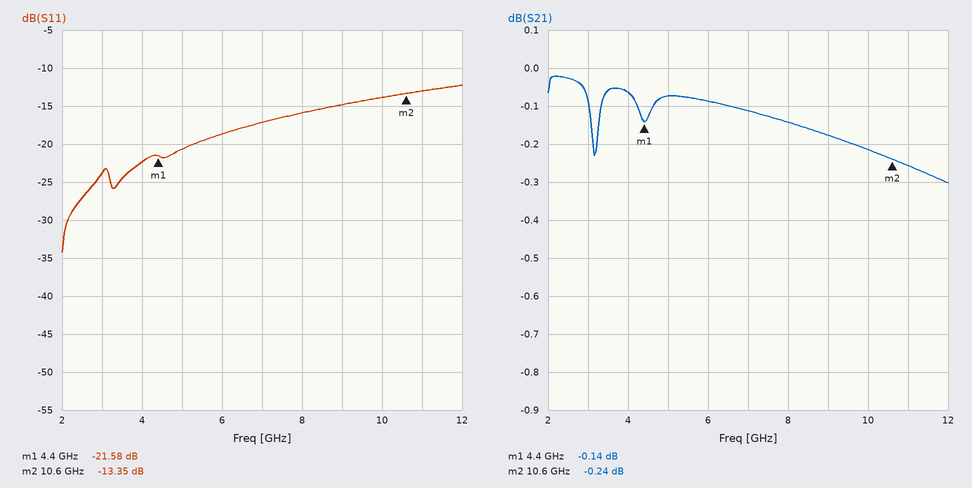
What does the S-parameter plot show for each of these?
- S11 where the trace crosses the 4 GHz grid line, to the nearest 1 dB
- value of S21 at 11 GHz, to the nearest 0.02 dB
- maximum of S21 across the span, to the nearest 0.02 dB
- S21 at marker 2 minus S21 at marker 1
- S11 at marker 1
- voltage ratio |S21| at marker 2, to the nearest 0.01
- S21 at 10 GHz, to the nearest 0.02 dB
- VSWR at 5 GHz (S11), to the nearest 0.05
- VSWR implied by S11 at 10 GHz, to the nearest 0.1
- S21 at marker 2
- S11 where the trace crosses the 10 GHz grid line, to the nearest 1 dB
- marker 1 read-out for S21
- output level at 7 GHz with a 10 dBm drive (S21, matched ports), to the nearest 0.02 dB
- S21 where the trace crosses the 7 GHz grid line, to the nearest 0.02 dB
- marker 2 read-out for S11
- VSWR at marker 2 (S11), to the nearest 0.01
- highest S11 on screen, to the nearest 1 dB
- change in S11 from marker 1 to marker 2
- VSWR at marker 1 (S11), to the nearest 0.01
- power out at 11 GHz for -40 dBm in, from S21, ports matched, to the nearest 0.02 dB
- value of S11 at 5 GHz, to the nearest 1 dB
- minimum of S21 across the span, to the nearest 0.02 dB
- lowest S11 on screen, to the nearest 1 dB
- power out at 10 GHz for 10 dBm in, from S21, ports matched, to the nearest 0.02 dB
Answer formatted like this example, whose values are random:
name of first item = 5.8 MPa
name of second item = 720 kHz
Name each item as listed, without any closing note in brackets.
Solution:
S11 where the trace crosses the 4 GHz grid line, to the nearest 1 dB = -22 dB
value of S21 at 11 GHz, to the nearest 0.02 dB = -0.26 dB
maximum of S21 across the span, to the nearest 0.02 dB = -0.02 dB
S21 at marker 2 minus S21 at marker 1 = -0.10 dB
S11 at marker 1 = -21.58 dB
voltage ratio |S21| at marker 2, to the nearest 0.01 = 0.97
S21 at 10 GHz, to the nearest 0.02 dB = -0.22 dB
VSWR at 5 GHz (S11), to the nearest 0.05 = 1.20
VSWR implied by S11 at 10 GHz, to the nearest 0.1 = 1.5
S21 at marker 2 = -0.24 dB
S11 where the trace crosses the 10 GHz grid line, to the nearest 1 dB = -14 dB
marker 1 read-out for S21 = -0.14 dB
output level at 7 GHz with a 10 dBm drive (S21, matched ports), to the nearest 0.02 dB = 9.88 dBm
S21 where the trace crosses the 7 GHz grid line, to the nearest 0.02 dB = -0.12 dB
marker 2 read-out for S11 = -13.35 dB
VSWR at marker 2 (S11), to the nearest 0.01 = 1.55
highest S11 on screen, to the nearest 1 dB = -12 dB
change in S11 from marker 1 to marker 2 = 8.23 dB
VSWR at marker 1 (S11), to the nearest 0.01 = 1.18
power out at 11 GHz for -40 dBm in, from S21, ports matched, to the nearest 0.02 dB = -40.26 dBm
value of S11 at 5 GHz, to the nearest 1 dB = -21 dB
minimum of S21 across the span, to the nearest 0.02 dB = -0.30 dB
lowest S11 on screen, to the nearest 1 dB = -34 dB
power out at 10 GHz for 10 dBm in, from S21, ports matched, to the nearest 0.02 dB = 9.78 dBm
